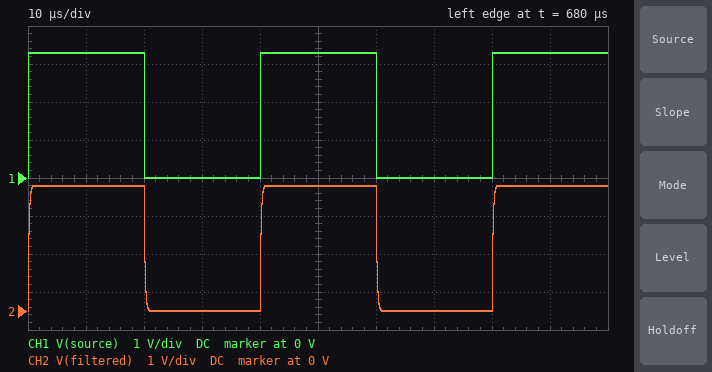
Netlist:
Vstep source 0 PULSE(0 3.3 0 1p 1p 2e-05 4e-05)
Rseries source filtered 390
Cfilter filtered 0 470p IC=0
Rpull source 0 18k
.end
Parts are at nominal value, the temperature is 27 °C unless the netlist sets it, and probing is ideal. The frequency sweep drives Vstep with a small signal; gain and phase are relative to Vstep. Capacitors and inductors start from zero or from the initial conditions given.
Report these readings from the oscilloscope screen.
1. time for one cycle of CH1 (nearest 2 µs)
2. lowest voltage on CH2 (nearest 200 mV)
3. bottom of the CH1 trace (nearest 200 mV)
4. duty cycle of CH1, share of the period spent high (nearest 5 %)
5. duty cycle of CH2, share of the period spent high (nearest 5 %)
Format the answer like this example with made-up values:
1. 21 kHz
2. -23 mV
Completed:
1. 40 µs
2. 0 V
3. 0 V
4. 50 %
5. 50 %
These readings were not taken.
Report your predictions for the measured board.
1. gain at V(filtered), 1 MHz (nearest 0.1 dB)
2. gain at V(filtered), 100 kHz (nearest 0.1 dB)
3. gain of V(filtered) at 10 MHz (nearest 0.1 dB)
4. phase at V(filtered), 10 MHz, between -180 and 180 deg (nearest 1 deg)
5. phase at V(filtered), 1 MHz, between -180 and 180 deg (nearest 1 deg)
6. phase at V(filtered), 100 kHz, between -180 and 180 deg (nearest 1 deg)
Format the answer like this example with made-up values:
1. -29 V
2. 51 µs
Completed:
1. -3.7 dB
2. -0.1 dB
3. -21.3 dB
4. -85 deg
5. -49 deg
6. -7 deg
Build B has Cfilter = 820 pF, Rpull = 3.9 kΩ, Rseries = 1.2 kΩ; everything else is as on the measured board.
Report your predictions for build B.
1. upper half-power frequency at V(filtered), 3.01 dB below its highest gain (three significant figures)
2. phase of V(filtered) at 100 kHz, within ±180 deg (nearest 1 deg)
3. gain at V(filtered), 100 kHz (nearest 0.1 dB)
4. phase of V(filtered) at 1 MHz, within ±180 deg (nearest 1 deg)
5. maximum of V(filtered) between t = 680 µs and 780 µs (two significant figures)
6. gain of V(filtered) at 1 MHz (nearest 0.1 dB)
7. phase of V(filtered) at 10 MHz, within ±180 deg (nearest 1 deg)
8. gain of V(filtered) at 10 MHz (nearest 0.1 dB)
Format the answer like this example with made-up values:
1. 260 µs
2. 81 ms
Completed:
1. 162 kHz
2. -32 deg
3. -1.4 dB
4. -81 deg
5. 3.3 V
6. -15.9 dB
7. -89 deg
8. -35.8 dB
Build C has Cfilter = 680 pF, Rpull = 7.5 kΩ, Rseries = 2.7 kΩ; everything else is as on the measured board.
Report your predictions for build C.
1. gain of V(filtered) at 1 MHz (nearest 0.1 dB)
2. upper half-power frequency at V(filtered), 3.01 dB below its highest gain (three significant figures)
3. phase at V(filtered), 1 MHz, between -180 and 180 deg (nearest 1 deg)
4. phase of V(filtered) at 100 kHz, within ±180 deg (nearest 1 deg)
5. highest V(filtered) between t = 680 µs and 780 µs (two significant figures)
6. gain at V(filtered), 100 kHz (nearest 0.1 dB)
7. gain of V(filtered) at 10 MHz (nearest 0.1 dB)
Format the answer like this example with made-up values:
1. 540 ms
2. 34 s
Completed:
1. -21.3 dB
2. 86.7 kHz
3. -85 deg
4. -49 deg
5. 3.3 V
6. -3.7 dB
7. -41.2 dB
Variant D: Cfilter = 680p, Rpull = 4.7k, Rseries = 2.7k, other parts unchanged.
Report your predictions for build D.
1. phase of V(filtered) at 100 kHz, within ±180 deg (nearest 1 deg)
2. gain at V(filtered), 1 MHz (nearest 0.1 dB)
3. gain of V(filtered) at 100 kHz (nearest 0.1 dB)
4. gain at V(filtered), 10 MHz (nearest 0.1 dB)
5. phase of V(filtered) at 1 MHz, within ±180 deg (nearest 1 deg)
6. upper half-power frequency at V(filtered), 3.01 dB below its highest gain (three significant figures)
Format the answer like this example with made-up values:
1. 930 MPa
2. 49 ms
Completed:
1. -49 deg
2. -21.3 dB
3. -3.7 dB
4. -41.2 dB
5. -85 deg
6. 86.7 kHz
